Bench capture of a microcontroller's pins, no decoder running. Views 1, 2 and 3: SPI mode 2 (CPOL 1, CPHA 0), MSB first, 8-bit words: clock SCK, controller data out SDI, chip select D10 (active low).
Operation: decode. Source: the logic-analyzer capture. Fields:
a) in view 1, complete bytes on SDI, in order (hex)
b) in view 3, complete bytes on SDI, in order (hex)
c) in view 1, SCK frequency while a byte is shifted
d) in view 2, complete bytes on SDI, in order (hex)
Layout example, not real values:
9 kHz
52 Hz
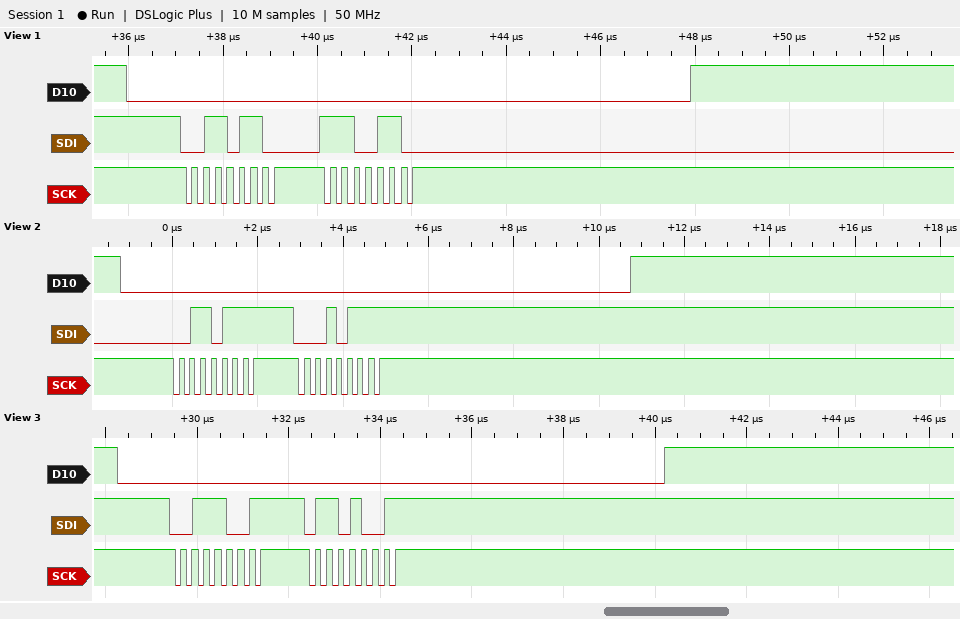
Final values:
36 E6
39 69
4 MHz
0x37 0x17
